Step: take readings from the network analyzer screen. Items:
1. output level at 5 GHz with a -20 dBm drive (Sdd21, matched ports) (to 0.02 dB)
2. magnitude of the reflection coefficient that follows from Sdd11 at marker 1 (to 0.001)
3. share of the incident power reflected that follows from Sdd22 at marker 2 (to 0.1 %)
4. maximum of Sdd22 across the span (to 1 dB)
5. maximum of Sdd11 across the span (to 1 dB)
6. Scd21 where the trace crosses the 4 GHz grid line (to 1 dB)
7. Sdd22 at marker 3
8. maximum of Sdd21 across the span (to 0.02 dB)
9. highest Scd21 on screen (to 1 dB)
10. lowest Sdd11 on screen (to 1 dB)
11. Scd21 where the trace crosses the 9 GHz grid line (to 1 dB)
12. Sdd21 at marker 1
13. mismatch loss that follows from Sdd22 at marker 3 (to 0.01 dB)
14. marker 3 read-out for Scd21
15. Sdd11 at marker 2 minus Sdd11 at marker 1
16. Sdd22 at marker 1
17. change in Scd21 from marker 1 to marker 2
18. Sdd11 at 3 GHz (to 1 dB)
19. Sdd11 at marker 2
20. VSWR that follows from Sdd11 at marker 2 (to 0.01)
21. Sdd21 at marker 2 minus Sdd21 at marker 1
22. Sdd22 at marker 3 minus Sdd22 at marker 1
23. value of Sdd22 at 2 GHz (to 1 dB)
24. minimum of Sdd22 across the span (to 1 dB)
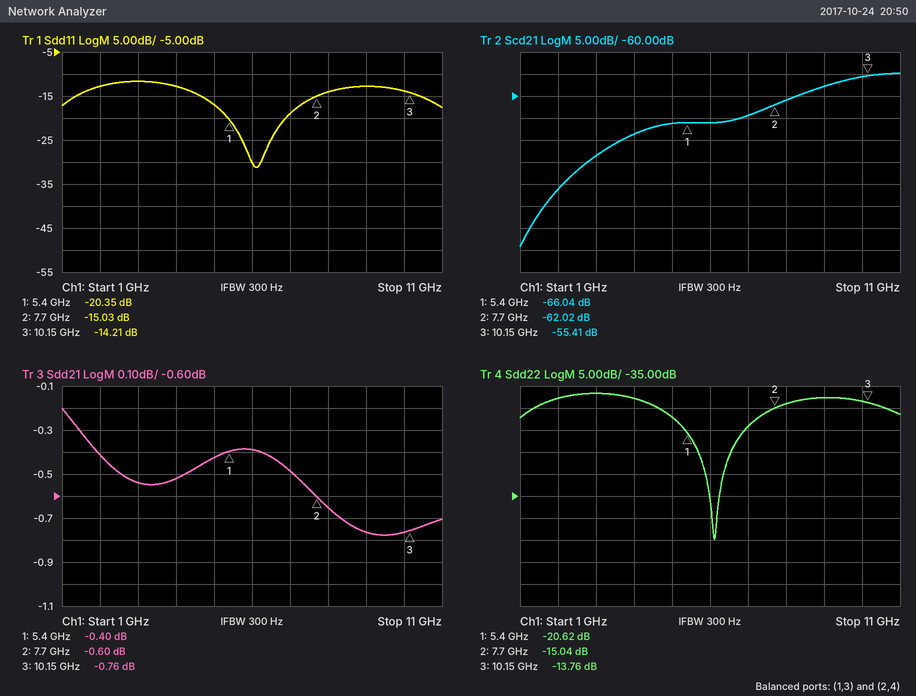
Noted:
-20.42 dBm
0.096
3.1 %
-12 dB
-12 dB
-69 dB
-13.76 dB
-0.20 dB
-55 dB
-31 dB
-58 dB
-0.40 dB
0.19 dB
-55.41 dB
5.32 dB
-20.62 dB
4.02 dB
-12 dB
-15.03 dB
1.43
-0.20 dB
6.86 dB
-13 dB
-45 dB
